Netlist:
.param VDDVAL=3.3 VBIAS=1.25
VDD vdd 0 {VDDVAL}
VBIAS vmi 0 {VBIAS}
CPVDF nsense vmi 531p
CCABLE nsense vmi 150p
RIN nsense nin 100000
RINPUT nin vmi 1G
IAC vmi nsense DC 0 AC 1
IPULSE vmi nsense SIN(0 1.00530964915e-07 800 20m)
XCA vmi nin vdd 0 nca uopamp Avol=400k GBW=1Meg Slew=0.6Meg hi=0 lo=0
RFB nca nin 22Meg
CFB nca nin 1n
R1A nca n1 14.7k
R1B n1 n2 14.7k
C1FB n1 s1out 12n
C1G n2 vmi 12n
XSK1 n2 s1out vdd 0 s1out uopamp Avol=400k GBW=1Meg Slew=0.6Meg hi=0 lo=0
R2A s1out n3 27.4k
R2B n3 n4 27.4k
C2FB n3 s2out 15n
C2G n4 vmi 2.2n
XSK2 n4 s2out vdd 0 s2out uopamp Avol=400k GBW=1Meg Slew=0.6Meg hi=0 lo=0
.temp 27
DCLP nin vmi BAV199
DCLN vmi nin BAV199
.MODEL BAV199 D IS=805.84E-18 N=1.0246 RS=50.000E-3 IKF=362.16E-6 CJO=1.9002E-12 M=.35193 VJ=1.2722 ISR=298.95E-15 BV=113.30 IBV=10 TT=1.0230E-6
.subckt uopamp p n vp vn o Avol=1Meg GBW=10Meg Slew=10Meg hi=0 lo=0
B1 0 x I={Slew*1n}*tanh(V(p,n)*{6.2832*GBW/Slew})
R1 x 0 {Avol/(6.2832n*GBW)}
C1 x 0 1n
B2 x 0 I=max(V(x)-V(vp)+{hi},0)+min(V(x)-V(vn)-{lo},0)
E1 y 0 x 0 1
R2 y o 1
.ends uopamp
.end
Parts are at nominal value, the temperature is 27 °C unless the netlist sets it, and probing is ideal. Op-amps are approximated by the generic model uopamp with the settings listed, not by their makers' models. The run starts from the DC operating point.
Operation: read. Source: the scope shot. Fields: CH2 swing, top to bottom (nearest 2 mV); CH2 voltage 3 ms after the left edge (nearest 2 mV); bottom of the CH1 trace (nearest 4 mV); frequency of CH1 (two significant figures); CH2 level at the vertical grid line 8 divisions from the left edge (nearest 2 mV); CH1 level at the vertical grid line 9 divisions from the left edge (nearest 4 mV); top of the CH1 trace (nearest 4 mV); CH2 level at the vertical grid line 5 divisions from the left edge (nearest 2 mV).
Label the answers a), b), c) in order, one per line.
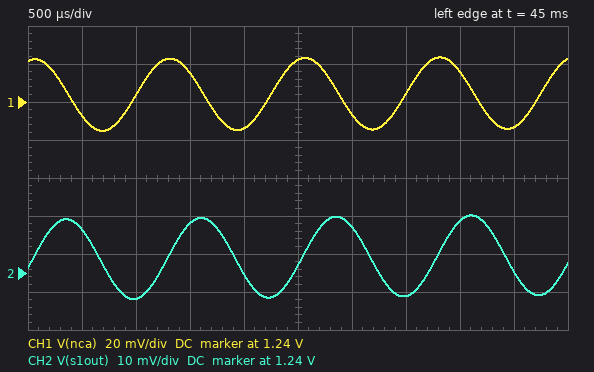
a) 22 mV
b) 1.252 V
c) 1.224 V
d) 800 Hz
e) 1.254 V
f) 1.228 V
g) 1.264 V
h) 1.242 V
